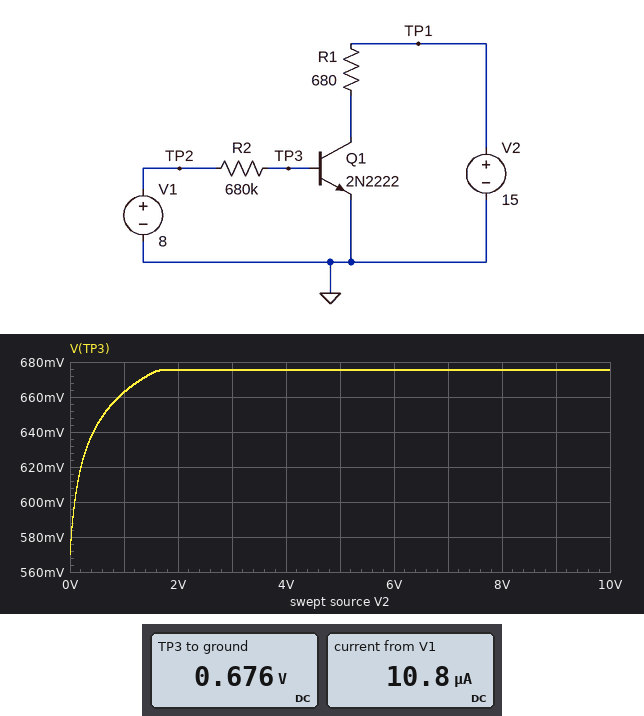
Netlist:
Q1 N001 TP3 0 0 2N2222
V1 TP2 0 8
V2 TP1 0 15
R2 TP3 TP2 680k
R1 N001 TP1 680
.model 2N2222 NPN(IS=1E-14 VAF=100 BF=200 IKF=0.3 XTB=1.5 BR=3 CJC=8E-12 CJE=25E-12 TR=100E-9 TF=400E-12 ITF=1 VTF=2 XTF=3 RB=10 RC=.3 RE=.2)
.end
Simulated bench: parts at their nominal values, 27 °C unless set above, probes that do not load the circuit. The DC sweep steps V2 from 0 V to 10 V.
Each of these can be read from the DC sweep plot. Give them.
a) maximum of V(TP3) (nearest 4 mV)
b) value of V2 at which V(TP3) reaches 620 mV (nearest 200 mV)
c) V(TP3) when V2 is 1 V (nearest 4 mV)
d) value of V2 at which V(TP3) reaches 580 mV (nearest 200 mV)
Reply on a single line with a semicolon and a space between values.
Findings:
676 mV; 200 mV; 664 mV; 0 V
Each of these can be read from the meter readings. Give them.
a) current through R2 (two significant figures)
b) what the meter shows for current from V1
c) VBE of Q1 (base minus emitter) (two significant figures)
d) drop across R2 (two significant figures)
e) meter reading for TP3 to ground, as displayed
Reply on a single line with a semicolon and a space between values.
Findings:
11 µA; 10.8 µA; 680 mV; 7.3 V; 0.676 V
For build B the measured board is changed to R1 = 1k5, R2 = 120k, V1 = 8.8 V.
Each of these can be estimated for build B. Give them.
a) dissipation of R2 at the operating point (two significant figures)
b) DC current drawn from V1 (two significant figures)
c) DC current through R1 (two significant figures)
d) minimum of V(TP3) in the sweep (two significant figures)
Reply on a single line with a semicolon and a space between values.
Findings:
540 µW; 67 µA; 9.9 mA; 620 mV
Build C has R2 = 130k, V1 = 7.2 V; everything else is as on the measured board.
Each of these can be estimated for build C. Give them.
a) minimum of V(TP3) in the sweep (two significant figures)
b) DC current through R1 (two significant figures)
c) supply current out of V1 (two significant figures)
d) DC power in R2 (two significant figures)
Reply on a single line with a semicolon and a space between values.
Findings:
610 mV; 10 mA; 50 µA; 320 µW
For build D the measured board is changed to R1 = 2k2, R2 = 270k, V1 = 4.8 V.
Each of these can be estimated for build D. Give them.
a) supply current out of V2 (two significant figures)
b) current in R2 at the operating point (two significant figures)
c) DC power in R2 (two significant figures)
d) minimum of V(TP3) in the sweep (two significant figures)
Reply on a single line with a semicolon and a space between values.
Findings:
3.2 mA; 15 µA; 63 µW; 580 mV
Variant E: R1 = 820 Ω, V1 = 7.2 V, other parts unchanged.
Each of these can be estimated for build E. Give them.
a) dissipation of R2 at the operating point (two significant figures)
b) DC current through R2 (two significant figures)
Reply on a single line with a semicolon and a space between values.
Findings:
63 µW; 9.6 µA
